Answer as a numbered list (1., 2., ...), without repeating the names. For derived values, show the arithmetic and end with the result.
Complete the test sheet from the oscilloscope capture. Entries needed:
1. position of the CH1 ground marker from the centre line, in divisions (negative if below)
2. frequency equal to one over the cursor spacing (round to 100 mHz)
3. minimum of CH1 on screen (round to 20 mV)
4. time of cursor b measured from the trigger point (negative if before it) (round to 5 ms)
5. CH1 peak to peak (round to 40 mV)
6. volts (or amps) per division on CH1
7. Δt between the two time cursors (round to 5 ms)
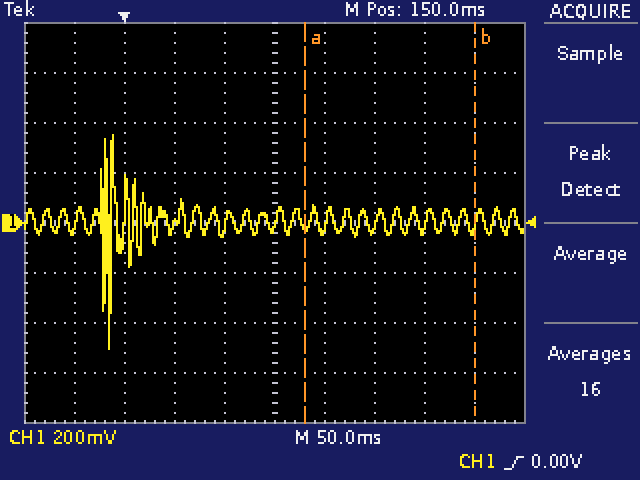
1. 0.0 div
2. 1 / 170 ms ≈ 5.9 Hz
3. -500 mV
4. +350 ms
5. 840 mV
6. 200 mV
7. 170 ms
